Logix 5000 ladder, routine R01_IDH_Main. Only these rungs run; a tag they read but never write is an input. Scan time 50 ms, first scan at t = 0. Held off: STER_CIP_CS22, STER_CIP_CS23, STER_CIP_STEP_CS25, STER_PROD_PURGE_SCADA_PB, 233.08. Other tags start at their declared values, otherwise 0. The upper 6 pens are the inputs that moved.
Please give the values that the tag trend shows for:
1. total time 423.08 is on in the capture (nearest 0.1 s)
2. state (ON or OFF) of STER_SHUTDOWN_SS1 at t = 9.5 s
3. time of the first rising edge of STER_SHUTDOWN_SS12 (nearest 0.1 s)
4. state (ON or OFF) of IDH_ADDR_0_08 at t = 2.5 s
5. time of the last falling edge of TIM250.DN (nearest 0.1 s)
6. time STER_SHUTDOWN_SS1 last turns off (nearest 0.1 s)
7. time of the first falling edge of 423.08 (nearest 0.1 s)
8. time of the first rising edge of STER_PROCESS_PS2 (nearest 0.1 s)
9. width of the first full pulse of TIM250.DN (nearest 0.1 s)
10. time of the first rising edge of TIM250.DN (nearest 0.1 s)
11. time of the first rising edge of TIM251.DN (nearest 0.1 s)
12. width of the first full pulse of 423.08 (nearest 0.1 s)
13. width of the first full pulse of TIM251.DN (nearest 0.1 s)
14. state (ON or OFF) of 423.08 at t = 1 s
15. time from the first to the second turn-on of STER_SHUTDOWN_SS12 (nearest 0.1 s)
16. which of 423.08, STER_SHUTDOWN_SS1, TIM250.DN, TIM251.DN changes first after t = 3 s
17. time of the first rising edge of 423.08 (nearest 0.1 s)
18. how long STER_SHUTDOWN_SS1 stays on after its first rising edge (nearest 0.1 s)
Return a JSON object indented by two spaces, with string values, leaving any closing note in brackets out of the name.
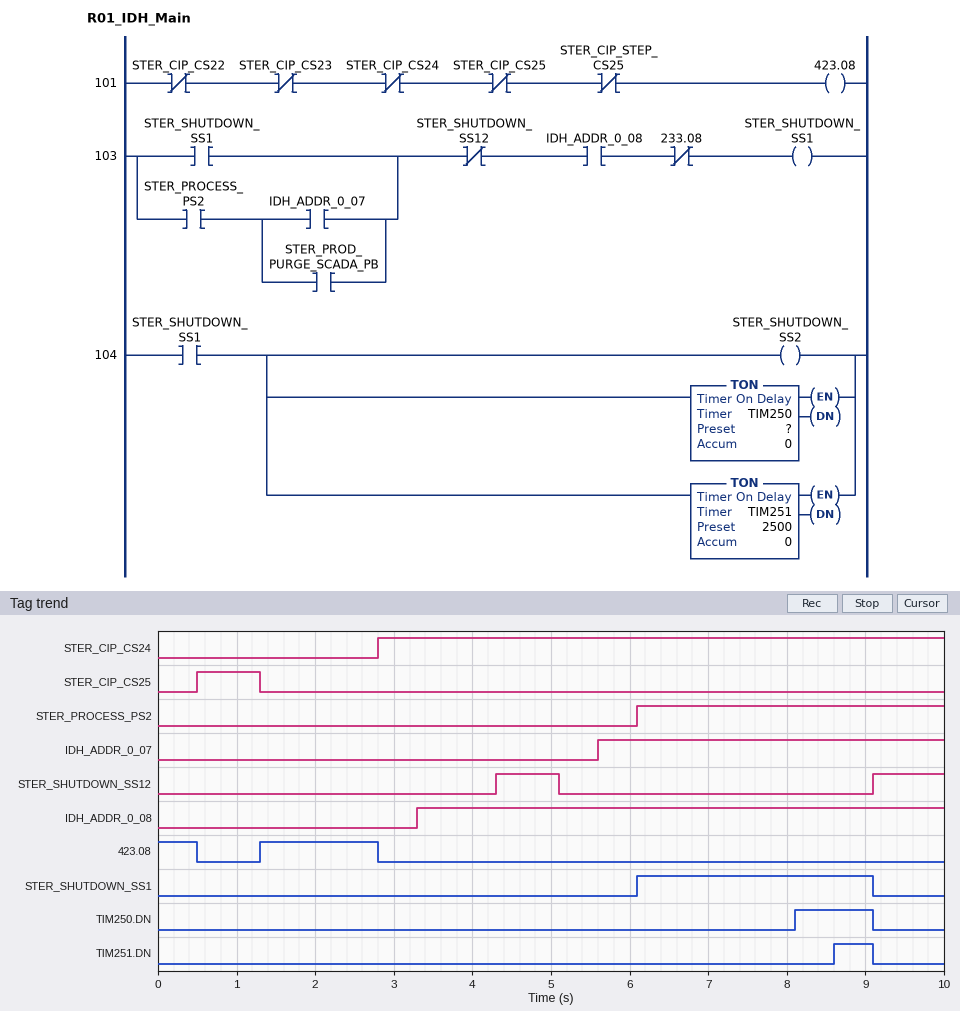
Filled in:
{
  "total time 423.08 is on in the capture": "2.0 s",
  "state (ON or OFF) of STER_SHUTDOWN_SS1 at t = 9.5 s": "OFF",
  "time of the first rising edge of STER_SHUTDOWN_SS12": "4.3 s",
  "state (ON or OFF) of IDH_ADDR_0_08 at t = 2.5 s": "OFF",
  "time of the last falling edge of TIM250.DN": "9.1 s",
  "time STER_SHUTDOWN_SS1 last turns off": "9.1 s",
  "time of the first falling edge of 423.08": "0.5 s",
  "time of the first rising edge of STER_PROCESS_PS2": "6.1 s",
  "width of the first full pulse of TIM250.DN": "1.0 s",
  "time of the first rising edge of TIM250.DN": "8.1 s",
  "time of the first rising edge of TIM251.DN": "8.6 s",
  "width of the first full pulse of 423.08": "1.5 s",
  "width of the first full pulse of TIM251.DN": "0.5 s",
  "state (ON or OFF) of 423.08 at t = 1 s": "OFF",
  "time from the first to the second turn-on of STER_SHUTDOWN_SS12": "4.8 s",
  "which of 423.08, STER_SHUTDOWN_SS1, TIM250.DN, TIM251.DN changes first after t = 3 s": "STER_SHUTDOWN_SS1",
  "time of the first rising edge of 423.08": "1.3 s",
  "how long STER_SHUTDOWN_SS1 stays on after its first rising edge": "3.0 s"
}
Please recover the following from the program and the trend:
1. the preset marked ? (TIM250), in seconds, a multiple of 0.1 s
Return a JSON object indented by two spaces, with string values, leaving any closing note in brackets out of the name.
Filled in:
{
  "the preset marked ? (TIM250), in seconds, a multiple of 0.1 s": "2.0 s"
}
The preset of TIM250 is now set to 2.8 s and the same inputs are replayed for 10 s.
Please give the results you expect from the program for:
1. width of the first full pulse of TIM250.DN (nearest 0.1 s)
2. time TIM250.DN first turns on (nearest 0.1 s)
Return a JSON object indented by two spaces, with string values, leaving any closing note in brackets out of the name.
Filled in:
{
  "width of the first full pulse of TIM250.DN": "0.2 s",
  "time TIM250.DN first turns on": "8.9 s"
}
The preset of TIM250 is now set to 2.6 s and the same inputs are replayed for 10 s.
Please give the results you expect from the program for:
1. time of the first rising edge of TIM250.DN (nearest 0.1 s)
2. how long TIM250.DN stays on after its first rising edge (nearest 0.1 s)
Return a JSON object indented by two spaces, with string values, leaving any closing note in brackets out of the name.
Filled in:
{
  "time of the first rising edge of TIM250.DN": "8.7 s",
  "how long TIM250.DN stays on after its first rising edge": "0.4 s"
}
